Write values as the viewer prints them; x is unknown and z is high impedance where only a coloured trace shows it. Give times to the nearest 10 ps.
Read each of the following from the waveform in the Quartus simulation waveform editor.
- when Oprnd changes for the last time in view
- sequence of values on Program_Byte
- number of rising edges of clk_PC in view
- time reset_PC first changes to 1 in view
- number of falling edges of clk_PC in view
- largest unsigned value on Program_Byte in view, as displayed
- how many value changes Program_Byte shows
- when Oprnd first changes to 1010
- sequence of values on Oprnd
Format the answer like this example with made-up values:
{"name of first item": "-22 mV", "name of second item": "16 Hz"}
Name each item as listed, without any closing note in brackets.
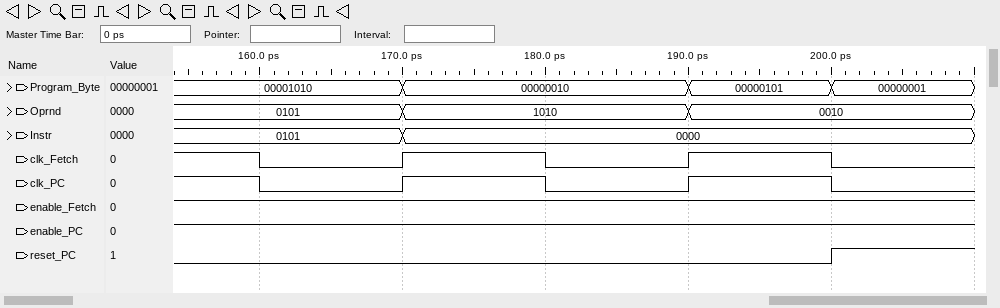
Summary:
{"when Oprnd changes for the last time in view": "190 ps", "sequence of values on Program_Byte": "00001010, 00000010, 00000101, 00000001", "number of rising edges of clk_PC in view": "2", "time reset_PC first changes to 1 in view": "200 ps", "number of falling edges of clk_PC in view": "3", "largest unsigned value on Program_Byte in view, as displayed": "00001010", "how many value changes Program_Byte shows": "3", "when Oprnd first changes to 1010": "170 ps", "sequence of values on Oprnd": "0101, 1010, 0010"}
